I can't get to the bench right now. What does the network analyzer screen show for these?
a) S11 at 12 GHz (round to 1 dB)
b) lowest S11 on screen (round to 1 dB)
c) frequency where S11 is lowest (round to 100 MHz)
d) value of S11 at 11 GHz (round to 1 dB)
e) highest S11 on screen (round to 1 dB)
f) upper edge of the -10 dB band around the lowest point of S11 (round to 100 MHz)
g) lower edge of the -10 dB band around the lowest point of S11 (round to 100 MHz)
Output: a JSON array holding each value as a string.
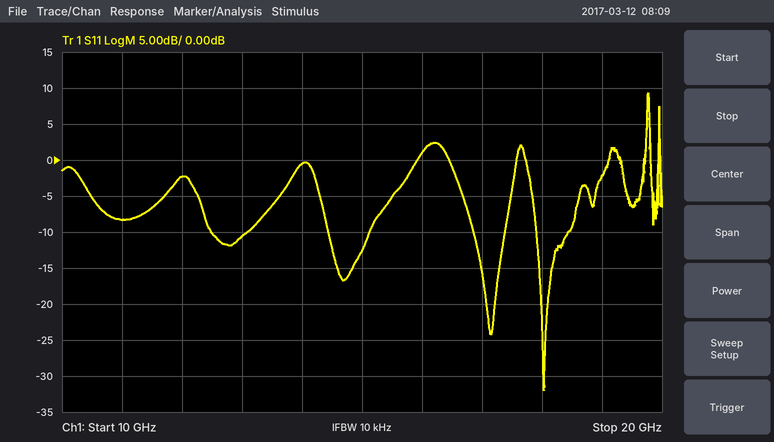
["-2 dB", "-32 dB", "18.0 GHz", "-8 dB", "9 dB", "18.4 GHz", "17.9 GHz"]
